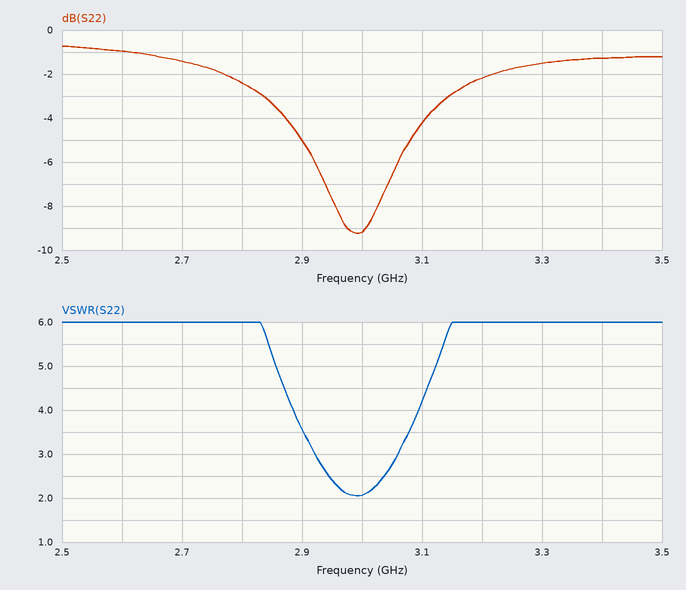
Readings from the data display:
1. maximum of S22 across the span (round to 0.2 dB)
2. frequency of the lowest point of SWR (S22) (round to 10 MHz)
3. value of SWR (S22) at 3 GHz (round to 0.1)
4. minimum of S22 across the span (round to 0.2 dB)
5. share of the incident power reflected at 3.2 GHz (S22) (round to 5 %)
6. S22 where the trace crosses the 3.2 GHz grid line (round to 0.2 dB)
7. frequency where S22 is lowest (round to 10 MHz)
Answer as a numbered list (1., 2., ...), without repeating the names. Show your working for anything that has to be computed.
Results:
1. -0.8 dB
2. 2.99 GHz
3. 2.1
4. -9.2 dB
5. 10^(-2.2/10) ≈ 60 %
6. -2.2 dB
7. 2.99 GHz
